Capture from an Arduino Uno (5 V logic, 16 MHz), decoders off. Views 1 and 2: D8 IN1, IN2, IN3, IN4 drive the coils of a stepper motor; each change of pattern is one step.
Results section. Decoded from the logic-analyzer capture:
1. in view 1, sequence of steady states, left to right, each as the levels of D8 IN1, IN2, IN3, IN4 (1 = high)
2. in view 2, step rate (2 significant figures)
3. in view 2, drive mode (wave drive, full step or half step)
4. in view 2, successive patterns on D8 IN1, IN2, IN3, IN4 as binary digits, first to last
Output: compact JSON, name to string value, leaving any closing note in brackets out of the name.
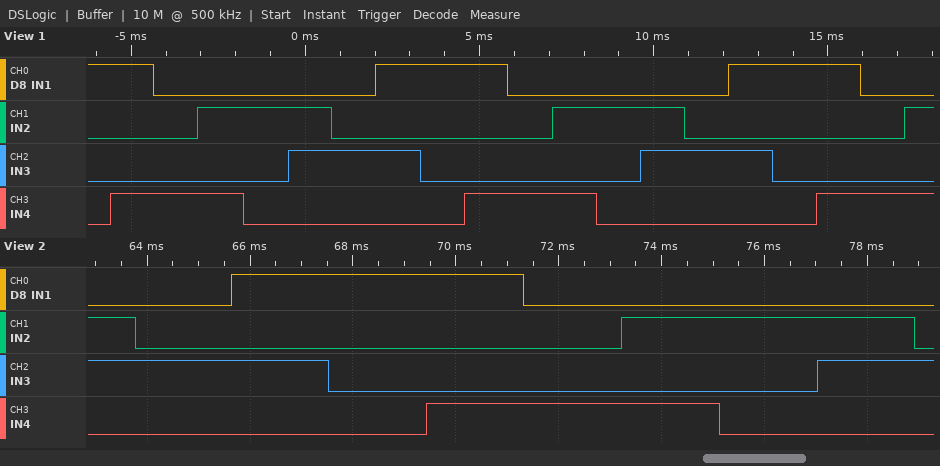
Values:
{"in view 1, sequence of steady states, left to right, each as the levels of D8 IN1, IN2, IN3, IN4": "1000 1001 0001 0101 0100 0110 0010 1010 1000 1001 0001 0101 0100 0110 0010 1010 1000 1001 0001 0101", "in view 2, step rate": "530 steps/s", "in view 2, drive mode": "half step", "in view 2, successive patterns on D8 IN1, IN2, IN3, IN4 as binary digits, first to last": "0110 0010 1010 1000 1001 0001 0101 0100 0110 0010"}
